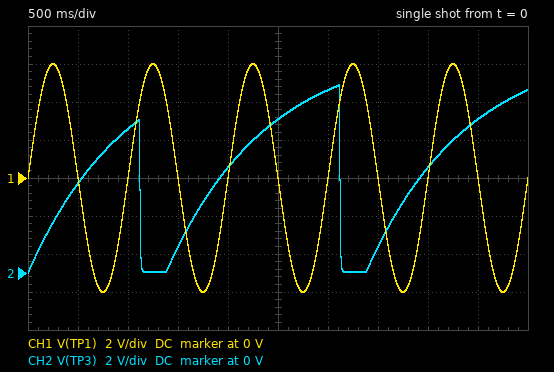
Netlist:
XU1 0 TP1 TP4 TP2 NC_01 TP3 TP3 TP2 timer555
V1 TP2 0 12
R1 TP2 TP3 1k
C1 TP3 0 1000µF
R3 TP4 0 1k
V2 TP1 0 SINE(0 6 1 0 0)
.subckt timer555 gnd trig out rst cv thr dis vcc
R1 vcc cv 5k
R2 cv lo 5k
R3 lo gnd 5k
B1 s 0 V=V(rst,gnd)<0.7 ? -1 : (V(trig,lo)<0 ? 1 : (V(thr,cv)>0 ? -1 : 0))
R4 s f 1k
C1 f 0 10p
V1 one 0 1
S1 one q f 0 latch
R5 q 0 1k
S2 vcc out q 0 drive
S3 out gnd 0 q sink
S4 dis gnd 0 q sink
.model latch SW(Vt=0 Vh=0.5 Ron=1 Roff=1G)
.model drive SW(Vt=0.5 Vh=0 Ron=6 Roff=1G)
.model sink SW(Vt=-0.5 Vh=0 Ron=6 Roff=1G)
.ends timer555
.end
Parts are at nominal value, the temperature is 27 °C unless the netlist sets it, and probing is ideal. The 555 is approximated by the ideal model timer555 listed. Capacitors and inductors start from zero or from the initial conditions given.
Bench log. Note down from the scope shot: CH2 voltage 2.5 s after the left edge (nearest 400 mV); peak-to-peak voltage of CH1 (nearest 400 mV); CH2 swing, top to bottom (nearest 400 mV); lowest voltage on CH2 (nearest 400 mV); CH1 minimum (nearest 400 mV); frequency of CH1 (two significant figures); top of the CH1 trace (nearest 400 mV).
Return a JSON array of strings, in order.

["8.0 V", "12.0 V", "10.0 V", "0 V", "-6.0 V", "1.0 Hz", "6.0 V"]
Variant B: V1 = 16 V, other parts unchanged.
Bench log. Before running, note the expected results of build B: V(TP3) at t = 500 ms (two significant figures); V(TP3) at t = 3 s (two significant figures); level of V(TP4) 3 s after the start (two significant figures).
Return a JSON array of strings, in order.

["6.3 V", "13 V", "16 V"]
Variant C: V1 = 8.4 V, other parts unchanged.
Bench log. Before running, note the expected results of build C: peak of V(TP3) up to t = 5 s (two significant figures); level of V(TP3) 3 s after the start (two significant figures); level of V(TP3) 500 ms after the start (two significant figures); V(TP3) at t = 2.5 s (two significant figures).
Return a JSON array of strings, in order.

["6.8 V", "6.7 V", "3.3 V", "5.6 V"]
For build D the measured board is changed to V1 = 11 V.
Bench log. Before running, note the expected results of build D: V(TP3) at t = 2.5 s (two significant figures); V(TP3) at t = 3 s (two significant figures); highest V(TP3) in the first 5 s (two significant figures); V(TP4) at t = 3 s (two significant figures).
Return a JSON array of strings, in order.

["7.4 V", "8.8 V", "9.0 V", "11 V"]
